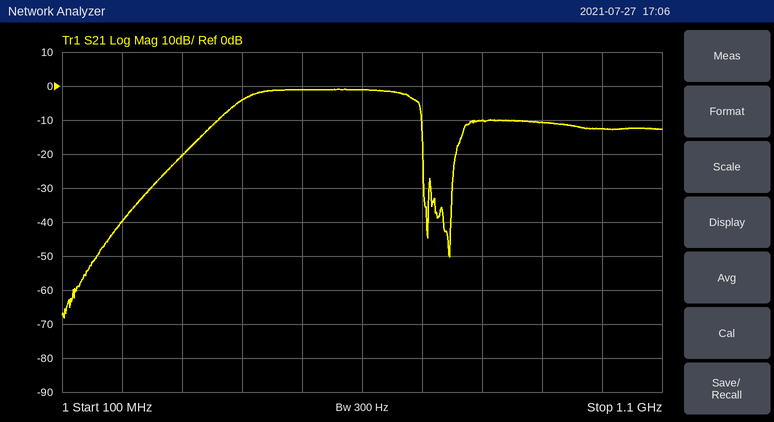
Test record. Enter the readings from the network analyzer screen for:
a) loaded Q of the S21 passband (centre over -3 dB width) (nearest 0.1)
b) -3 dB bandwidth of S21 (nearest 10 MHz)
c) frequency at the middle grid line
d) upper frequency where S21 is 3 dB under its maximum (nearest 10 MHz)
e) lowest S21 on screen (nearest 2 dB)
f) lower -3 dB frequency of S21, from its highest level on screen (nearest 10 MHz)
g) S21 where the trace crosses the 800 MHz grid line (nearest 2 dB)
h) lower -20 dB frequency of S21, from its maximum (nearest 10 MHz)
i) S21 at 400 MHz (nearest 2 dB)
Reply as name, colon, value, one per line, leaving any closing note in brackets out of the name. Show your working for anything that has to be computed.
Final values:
loaded Q of the S21 passband (centre over -3 dB width): 545 MHz / 290 MHz ≈ 1.9
-3 dB bandwidth of S21: 690 MHz − 400 MHz = 290 MHz
frequency at the middle grid line: 600 MHz
upper frequency where S21 is 3 dB under its maximum: 690 MHz
lowest S21 on screen: -68 dB
lower -3 dB frequency of S21, from its highest level on screen: 400 MHz
S21 where the trace crosses the 800 MHz grid line: -10 dB
lower -20 dB frequency of S21, from its maximum: 300 MHz
S21 at 400 MHz: -4 dB
